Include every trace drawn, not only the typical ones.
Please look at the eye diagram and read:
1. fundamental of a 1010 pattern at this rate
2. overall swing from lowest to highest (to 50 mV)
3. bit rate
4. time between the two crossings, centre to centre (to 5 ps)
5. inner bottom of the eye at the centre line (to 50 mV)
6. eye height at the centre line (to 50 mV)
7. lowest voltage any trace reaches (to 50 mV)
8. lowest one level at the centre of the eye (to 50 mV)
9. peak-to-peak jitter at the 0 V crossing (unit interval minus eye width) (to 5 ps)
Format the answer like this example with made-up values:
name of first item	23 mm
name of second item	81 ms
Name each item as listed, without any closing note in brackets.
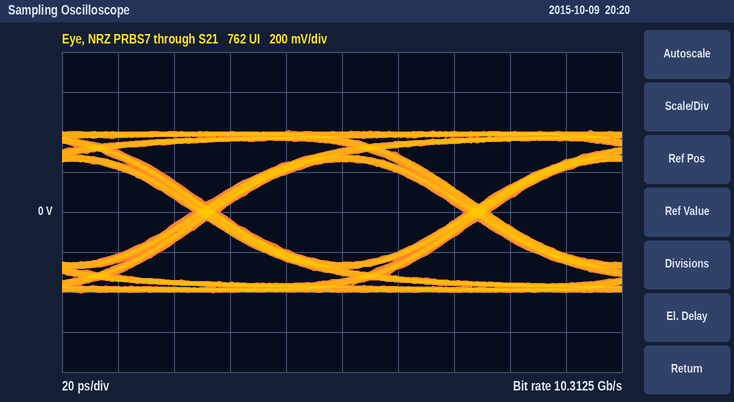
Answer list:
fundamental of a 1010 pattern at this rate	5.15625 GHz
overall swing from lowest to highest	800 mV
bit rate	10.3125 Gb/s
time between the two crossings, centre to centre	95 ps
inner bottom of the eye at the centre line	-250 mV
eye height at the centre line	500 mV
lowest voltage any trace reaches	-400 mV
lowest one level at the centre of the eye	250 mV
peak-to-peak jitter at the 0 V crossing (unit interval minus eye width)	10 ps
